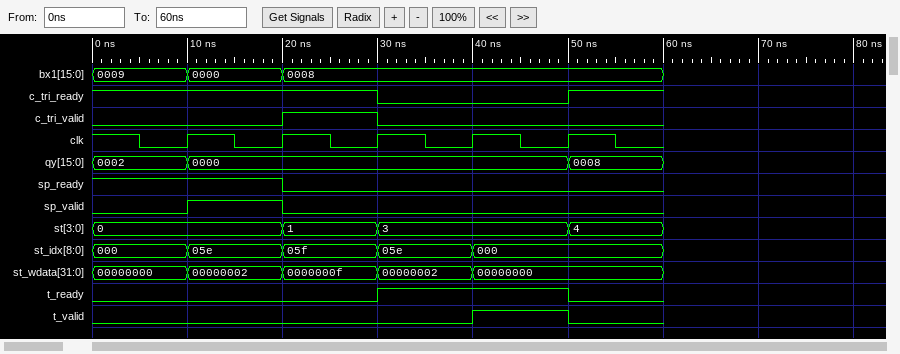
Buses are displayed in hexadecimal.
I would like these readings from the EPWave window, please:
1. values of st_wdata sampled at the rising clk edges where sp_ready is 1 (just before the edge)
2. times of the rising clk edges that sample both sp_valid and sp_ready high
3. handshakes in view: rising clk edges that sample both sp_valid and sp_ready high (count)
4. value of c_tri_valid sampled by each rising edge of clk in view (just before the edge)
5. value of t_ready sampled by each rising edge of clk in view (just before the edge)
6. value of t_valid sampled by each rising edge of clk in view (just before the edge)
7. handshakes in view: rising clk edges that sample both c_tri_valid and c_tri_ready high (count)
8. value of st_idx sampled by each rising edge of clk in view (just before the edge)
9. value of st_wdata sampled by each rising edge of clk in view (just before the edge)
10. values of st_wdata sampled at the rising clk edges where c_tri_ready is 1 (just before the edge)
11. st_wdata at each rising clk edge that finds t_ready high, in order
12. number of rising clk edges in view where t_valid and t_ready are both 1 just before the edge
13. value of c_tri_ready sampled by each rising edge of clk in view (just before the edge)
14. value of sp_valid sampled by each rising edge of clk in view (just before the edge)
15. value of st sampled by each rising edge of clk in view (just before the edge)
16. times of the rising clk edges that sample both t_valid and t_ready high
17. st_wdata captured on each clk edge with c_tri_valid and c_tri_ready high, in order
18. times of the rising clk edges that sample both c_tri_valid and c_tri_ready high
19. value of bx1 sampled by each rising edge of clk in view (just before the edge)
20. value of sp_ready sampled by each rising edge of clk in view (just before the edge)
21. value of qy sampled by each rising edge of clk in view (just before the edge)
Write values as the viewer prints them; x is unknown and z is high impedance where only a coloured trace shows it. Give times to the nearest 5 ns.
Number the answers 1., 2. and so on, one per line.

1. 00000000, 00000002
2. 20 ns
3. 1
4. 0 0 1 0 0
5. 0 0 0 1 1
6. 0 0 0 0 1
7. 1
8. 000, 05e, 05f, 05e, 000
9. 00000000, 00000002, 0000000f, 00000002, 00000000
10. 00000000, 00000002, 0000000f
11. 00000002, 00000000
12. 1
13. 1 1 1 0 0
14. 0 1 0 0 0
15. 0, 0, 1, 3, 3
16. 50 ns
17. 0000000f
18. 30 ns
19. 0009, 0000, 0008, 0008, 0008
20. 1 1 0 0 0
21. 0002, 0000, 0000, 0000, 0000
